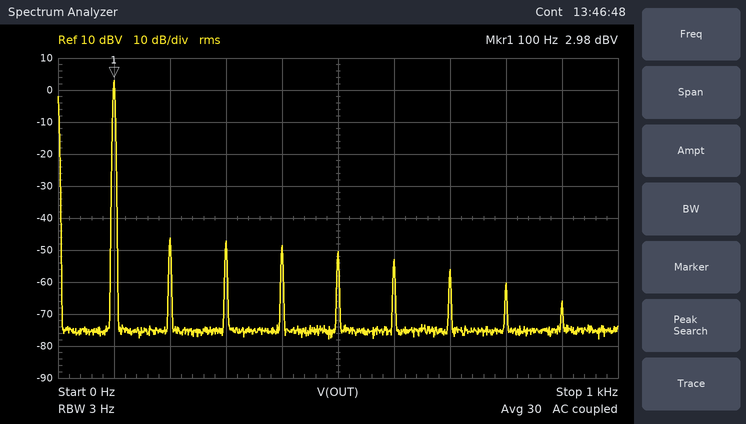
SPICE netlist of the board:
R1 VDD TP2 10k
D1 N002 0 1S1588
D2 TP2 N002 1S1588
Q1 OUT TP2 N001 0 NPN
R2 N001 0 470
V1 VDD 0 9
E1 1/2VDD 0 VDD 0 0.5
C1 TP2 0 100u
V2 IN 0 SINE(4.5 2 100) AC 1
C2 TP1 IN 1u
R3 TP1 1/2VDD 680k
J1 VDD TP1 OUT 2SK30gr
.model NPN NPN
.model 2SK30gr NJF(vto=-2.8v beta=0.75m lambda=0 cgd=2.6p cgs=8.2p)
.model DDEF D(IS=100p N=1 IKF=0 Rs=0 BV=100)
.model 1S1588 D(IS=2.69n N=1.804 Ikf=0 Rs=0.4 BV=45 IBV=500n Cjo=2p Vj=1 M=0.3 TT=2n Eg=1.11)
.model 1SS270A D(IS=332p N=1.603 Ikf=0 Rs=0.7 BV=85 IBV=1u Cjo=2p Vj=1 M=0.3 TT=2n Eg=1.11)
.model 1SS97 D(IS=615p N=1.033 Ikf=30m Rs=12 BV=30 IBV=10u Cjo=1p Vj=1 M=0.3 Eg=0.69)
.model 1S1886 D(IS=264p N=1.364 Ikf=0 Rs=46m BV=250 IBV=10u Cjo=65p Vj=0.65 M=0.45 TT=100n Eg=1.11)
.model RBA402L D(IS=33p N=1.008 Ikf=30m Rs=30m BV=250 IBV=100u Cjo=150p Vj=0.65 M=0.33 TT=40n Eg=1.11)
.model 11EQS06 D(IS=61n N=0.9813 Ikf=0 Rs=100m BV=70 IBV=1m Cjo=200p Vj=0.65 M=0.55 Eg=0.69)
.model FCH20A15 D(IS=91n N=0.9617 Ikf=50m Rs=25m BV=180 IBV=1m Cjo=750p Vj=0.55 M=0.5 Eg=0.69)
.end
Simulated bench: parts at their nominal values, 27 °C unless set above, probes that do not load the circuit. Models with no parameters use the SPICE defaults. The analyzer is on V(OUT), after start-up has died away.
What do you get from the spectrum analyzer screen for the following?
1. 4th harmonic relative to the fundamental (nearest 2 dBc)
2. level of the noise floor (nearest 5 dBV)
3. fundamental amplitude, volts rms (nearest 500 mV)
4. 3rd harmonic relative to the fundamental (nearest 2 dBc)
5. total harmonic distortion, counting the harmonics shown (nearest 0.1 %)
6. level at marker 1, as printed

-52 dBc
-75 dBV
1.5 V
-50 dBc
0.6 %
2.98 dBV
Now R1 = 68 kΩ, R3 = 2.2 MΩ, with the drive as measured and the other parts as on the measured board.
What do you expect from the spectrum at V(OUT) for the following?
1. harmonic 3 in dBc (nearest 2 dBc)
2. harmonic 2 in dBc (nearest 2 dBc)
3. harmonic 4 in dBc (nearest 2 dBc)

-48 dBc
-46 dBc
-50 dBc
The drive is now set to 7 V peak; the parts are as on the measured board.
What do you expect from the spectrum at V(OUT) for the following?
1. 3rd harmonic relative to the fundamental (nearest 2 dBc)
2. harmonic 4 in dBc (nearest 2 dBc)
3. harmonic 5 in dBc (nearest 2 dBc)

-16 dBc
-48 dBc
-40 dBc
